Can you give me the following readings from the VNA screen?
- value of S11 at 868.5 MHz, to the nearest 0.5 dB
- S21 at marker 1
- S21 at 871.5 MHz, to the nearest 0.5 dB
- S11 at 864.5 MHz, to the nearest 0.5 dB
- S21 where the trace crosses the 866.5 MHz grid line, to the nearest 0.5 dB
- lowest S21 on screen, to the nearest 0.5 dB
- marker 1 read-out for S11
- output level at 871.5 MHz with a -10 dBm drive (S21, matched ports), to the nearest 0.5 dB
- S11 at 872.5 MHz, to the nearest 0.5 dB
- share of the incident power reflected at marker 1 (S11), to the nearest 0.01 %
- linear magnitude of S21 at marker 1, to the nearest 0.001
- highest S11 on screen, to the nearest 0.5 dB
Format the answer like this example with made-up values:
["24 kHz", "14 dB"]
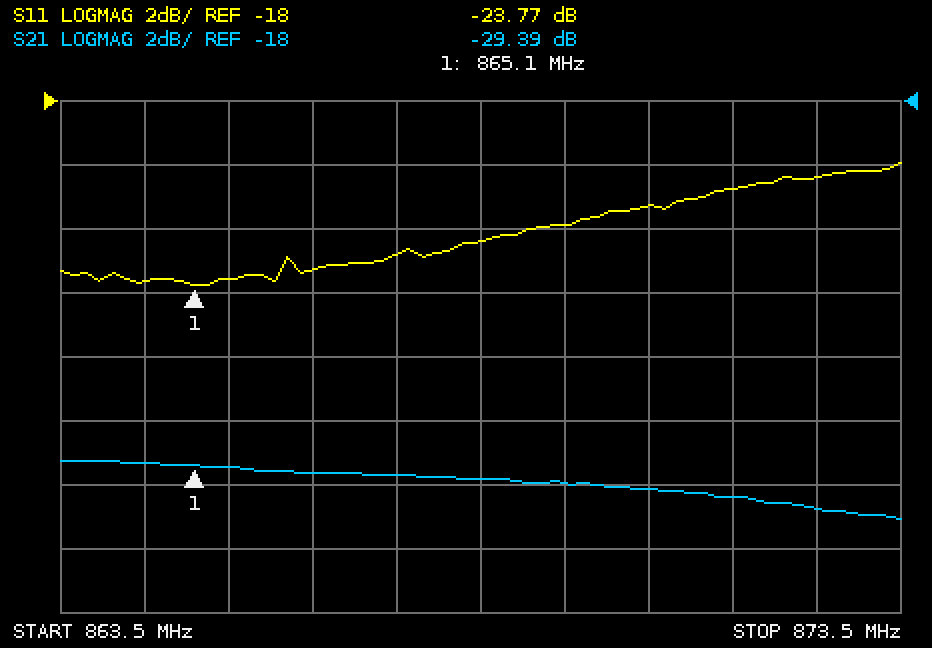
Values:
["-22.5 dB", "-29.39 dB", "-30.5 dB", "-23.5 dB", "-29.5 dB", "-31.0 dB", "-23.77 dB", "-40.5 dBm", "-20.5 dB", "0.42 %", "0.034", "-20.0 dB"]
